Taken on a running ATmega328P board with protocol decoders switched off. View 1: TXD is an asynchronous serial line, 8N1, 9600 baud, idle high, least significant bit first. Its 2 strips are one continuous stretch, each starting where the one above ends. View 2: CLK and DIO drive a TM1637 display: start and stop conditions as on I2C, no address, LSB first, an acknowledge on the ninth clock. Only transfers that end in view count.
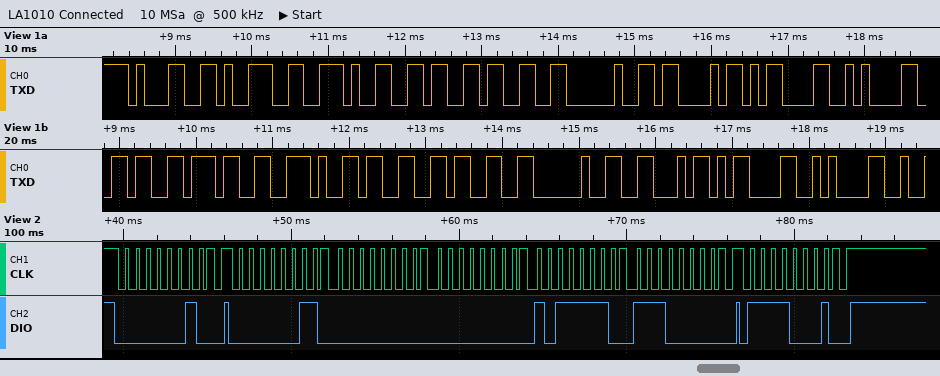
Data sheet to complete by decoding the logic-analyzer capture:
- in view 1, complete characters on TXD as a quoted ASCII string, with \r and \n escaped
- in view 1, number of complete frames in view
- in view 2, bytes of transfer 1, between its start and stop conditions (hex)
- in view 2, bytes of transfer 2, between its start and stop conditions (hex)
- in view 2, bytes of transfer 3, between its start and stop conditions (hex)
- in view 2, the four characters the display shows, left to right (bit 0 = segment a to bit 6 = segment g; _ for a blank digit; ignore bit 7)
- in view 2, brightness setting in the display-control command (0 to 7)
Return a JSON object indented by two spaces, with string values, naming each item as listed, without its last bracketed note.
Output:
{
  "in view 1, complete characters on TXD as a quoted ASCII string, with \\r and \\n escaped": "\"19.63 C\\r\\n67.33 F\\r\\n\"",
  "in view 1, number of complete frames in view": "18",
  "in view 2, bytes of transfer 1, between its start and stop conditions": "40",
  "in view 2, bytes of transfer 2, between its start and stop conditions": "C0 00 00 7D 07",
  "in view 2, bytes of transfer 3, between its start and stop conditions": "8F",
  "in view 2, the four characters the display shows, left to right": "__67",
  "in view 2, brightness setting in the display-control command": "7"
}
